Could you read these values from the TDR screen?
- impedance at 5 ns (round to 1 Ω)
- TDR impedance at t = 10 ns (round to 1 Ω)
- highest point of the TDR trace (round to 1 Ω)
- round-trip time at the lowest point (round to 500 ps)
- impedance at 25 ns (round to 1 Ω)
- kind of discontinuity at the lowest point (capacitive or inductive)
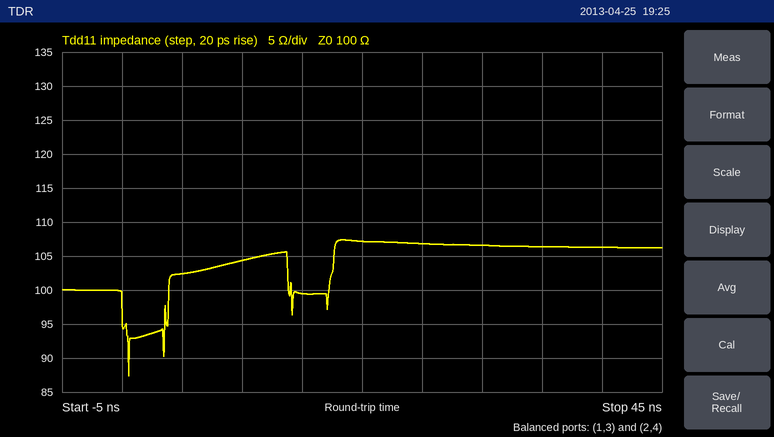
102 Ω
104 Ω
107 Ω
500 ps
107 Ω
capacitive
